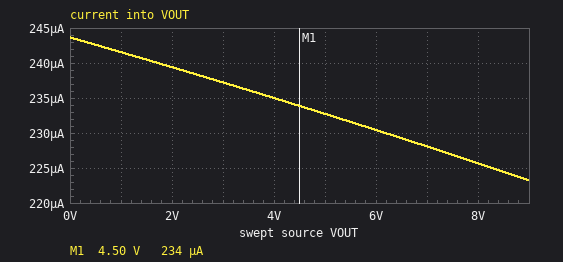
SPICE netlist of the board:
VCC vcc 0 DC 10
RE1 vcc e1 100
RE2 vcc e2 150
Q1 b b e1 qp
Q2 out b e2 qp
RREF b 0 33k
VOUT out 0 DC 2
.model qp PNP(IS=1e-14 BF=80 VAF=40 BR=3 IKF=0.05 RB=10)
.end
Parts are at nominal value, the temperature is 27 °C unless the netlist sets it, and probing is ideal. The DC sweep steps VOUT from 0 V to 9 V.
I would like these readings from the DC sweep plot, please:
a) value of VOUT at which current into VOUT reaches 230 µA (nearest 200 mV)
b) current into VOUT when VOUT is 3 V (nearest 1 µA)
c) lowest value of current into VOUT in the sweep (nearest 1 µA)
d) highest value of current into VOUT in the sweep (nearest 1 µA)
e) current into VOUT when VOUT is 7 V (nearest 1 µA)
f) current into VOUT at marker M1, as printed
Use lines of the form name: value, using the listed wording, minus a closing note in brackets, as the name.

value of VOUT at which current into VOUT reaches 230 µA: 6.2 V
current into VOUT when VOUT is 3 V: 237 µA
lowest value of current into VOUT in the sweep: 223 µA
highest value of current into VOUT in the sweep: 244 µA
current into VOUT when VOUT is 7 V: 228 µA
current into VOUT at marker M1, as printed: 234 µA
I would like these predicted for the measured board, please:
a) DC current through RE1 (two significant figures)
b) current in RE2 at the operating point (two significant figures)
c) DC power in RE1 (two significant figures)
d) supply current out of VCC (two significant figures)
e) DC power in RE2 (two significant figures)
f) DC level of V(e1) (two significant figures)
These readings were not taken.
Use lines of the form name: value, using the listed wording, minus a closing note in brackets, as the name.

DC current through RE1: 280 µA
current in RE2 at the operating point: 240 µA
DC power in RE1: 7.9 µW
supply current out of VCC: 520 µA
DC power in RE2: 8.8 µW
DC level of V(e1): 10 V
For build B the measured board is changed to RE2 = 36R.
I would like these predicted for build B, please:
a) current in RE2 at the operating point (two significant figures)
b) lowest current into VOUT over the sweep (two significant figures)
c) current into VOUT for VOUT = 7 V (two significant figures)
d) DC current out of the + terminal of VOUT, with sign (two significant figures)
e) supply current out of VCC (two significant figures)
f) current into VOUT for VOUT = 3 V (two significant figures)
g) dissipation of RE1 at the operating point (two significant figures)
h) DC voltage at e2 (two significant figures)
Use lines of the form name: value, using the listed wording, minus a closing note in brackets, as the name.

current in RE2 at the operating point: 490 µA
lowest current into VOUT over the sweep: 440 µA
current into VOUT for VOUT = 7 V: 450 µA
DC current out of the + terminal of VOUT, with sign: -480 µA
supply current out of VCC: 770 µA
current into VOUT for VOUT = 3 V: 480 µA
dissipation of RE1 at the operating point: 7.7 µW
DC voltage at e2: 10 V
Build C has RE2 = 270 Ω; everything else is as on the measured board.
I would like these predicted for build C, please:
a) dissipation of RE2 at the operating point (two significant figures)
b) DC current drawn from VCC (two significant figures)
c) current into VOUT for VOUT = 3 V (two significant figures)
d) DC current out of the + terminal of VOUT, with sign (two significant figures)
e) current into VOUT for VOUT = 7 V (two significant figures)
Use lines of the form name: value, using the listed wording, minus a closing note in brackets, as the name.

dissipation of RE2 at the operating point: 7.7 µW
DC current drawn from VCC: 450 µA
current into VOUT for VOUT = 3 V: 170 µA
DC current out of the + terminal of VOUT, with sign: -170 µA
current into VOUT for VOUT = 7 V: 160 µA
